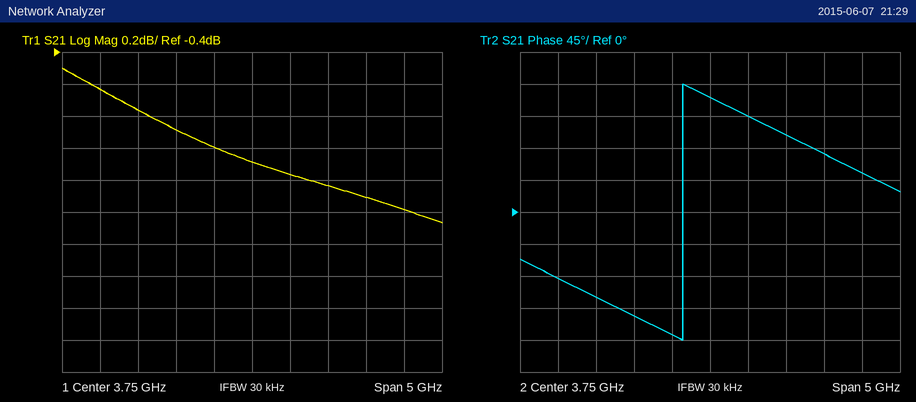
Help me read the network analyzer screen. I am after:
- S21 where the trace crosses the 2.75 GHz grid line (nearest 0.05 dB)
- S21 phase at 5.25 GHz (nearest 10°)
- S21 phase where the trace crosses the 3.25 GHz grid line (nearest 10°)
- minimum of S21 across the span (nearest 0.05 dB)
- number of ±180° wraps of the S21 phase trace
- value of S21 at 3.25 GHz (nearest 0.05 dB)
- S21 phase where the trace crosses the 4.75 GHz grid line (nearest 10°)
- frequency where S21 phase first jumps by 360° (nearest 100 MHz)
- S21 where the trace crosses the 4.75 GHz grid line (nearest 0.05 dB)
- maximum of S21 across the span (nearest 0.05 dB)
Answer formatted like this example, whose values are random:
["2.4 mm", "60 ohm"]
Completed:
["-0.90 dB", "80°", "-170°", "-1.45 dB", "1", "-1.00 dB", "110°", "3.4 GHz", "-1.25 dB", "-0.50 dB"]
